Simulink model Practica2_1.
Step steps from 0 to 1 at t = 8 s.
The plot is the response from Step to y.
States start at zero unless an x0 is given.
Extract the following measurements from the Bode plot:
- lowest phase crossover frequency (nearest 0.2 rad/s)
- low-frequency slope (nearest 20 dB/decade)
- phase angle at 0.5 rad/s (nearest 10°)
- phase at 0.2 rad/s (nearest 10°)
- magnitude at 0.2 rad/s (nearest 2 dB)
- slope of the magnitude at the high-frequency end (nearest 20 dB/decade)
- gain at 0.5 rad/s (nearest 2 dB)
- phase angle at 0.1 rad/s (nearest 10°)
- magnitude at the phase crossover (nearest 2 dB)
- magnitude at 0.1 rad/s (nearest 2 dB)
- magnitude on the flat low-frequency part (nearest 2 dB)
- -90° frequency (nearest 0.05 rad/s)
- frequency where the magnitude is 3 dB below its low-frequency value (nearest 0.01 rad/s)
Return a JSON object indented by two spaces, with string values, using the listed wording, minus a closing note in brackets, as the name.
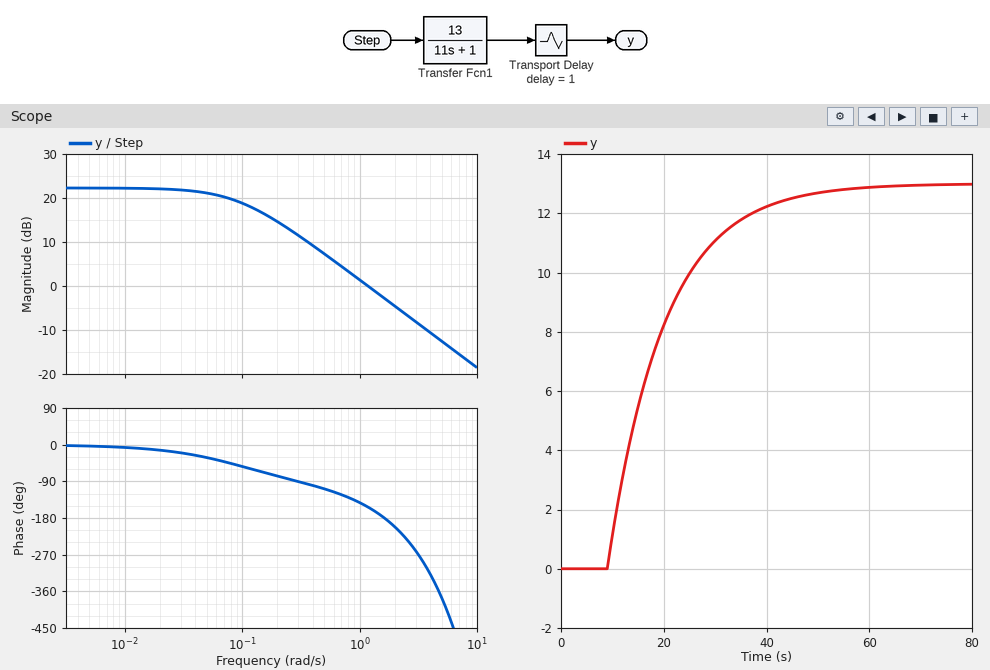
{
  "lowest phase crossover frequency": "1.6 rad/s",
  "low-frequency slope": "0 dB/decade",
  "phase angle at 0.5 rad/s": "-110°",
  "phase at 0.2 rad/s": "-80°",
  "magnitude at 0.2 rad/s": "14 dB",
  "slope of the magnitude at the high-frequency end": "-20 dB/decade",
  "gain at 0.5 rad/s": "8 dB",
  "phase angle at 0.1 rad/s": "-50°",
  "magnitude at the phase crossover": "-2 dB",
  "magnitude at 0.1 rad/s": "18 dB",
  "magnitude on the flat low-frequency part": "22 dB",
  "-90° frequency": "0.30 rad/s",
  "frequency where the magnitude is 3 dB below its low-frequency value": "0.09 rad/s"
}
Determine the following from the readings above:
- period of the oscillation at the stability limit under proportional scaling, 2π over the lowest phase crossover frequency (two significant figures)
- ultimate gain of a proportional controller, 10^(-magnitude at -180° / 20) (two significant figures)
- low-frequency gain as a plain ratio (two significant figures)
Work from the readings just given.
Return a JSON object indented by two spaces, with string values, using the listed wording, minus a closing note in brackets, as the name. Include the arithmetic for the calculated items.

{
  "period of the oscillation at the stability limit under proportional scaling, 2π over the lowest phase crossover frequency": "2π / 1.6 = 3.9 s",
  "ultimate gain of a proportional controller, 10^(-magnitude at -180° / 20)": "10^(2 / 20) = 1.3",
  "low-frequency gain as a plain ratio": "10^(22 / 20) = 13"
}
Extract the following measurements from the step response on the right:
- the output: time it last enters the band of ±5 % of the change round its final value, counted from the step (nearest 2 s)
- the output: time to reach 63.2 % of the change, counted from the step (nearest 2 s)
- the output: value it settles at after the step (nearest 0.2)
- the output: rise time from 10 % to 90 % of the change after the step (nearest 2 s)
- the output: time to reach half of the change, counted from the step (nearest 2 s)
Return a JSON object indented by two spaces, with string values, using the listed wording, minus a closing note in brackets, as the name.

{
  "the output: time it last enters the band of ±5 % of the change round its final value, counted from the step": "34 s",
  "the output: time to reach 63.2 % of the change, counted from the step": "12 s",
  "the output: value it settles at after the step": "13.0",
  "the output: rise time from 10 % to 90 % of the change after the step": "24 s",
  "the output: time to reach half of the change, counted from the step": "8 s"
}
